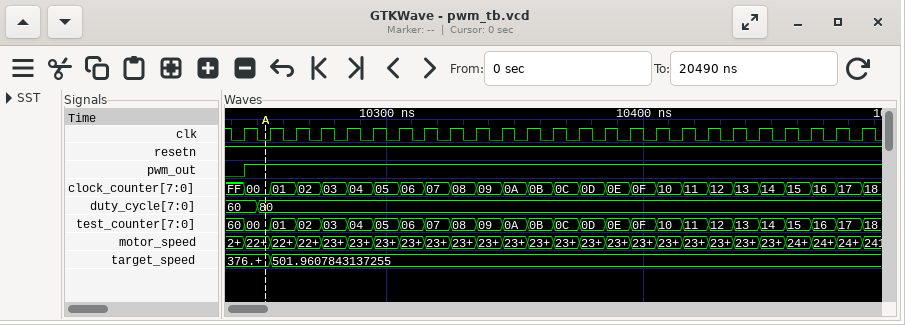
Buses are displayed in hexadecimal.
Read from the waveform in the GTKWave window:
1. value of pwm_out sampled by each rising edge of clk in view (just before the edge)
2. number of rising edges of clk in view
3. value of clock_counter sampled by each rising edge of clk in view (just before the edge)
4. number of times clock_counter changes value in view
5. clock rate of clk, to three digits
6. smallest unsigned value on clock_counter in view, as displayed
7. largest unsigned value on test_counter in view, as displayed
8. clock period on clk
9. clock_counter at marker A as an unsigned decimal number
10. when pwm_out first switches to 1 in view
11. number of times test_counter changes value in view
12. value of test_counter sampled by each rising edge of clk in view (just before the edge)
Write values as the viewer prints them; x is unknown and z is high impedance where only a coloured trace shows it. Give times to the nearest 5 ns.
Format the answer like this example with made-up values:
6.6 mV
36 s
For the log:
0 1 1 1 1 1 1 1 1 1 1 1 1 1 1 1 1 1 1 1 1 1 1 1 1
25
FF, 00, 01, 02, 03, 04, 05, 06, 07, 08, 09, 0A, 0B, 0C, 0D, 0E, 0F, 10, 11, 12, 13, 14, 15, 16, 17
25
100 MHz
00
60
10 ns
0
10245 ns
25
60, 00, 01, 02, 03, 04, 05, 06, 07, 08, 09, 0A, 0B, 0C, 0D, 0E, 0F, 10, 11, 12, 13, 14, 15, 16, 17
